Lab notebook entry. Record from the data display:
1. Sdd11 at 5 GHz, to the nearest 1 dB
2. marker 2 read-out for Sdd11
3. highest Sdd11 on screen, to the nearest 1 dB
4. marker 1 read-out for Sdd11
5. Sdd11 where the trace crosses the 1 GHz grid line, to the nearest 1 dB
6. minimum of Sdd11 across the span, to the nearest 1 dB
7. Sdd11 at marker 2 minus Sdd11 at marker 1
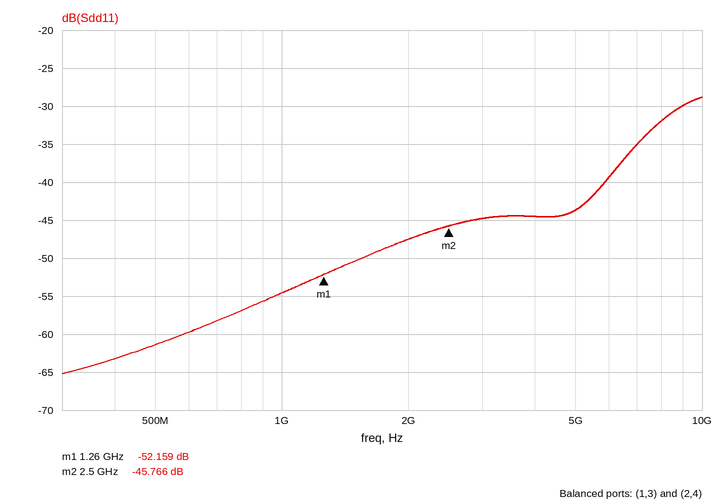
-44 dB
-45.766 dB
-29 dB
-52.159 dB
-55 dB
-65 dB
6.393 dB
